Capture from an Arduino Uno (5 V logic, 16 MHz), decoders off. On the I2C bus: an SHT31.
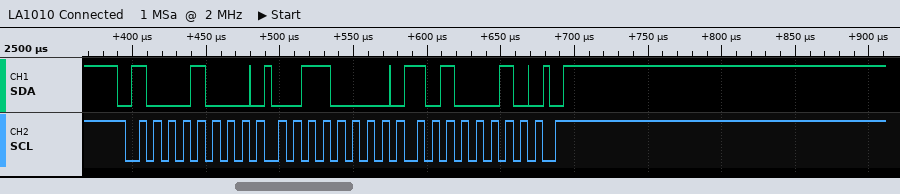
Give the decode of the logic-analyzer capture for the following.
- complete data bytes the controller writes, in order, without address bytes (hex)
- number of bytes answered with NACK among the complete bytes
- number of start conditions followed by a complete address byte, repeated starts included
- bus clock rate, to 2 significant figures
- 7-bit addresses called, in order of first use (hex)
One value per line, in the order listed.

30 A2
0
1
100 kHz
0x44
